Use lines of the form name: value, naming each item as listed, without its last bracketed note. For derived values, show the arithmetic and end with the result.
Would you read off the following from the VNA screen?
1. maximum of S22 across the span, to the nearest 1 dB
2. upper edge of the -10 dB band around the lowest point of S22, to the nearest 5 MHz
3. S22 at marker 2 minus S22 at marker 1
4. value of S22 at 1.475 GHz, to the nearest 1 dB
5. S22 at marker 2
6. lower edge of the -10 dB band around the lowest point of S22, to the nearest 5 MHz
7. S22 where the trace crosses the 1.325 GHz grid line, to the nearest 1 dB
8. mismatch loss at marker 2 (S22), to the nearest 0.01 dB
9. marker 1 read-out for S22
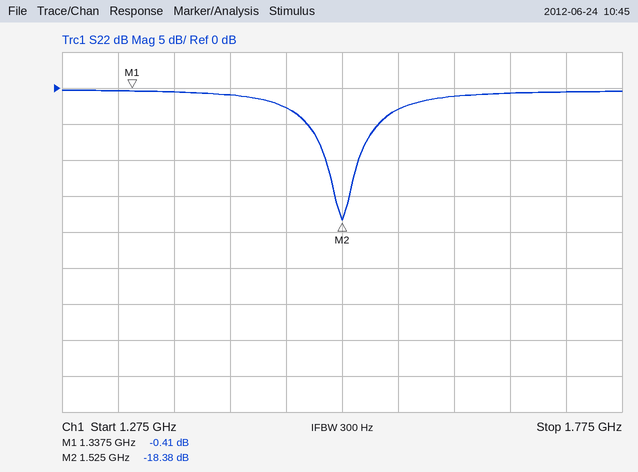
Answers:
maximum of S22 across the span, to the nearest 1 dB: 0 dB
upper edge of the -10 dB band around the lowest point of S22, to the nearest 5 MHz: 1.540 GHz
S22 at marker 2 minus S22 at marker 1: -18.38 − (-0.41) = -17.97 dB
value of S22 at 1.475 GHz, to the nearest 1 dB: -3 dB
S22 at marker 2: -18.38 dB
lower edge of the -10 dB band around the lowest point of S22, to the nearest 5 MHz: 1.510 GHz
S22 where the trace crosses the 1.325 GHz grid line, to the nearest 1 dB: 0 dB
mismatch loss at marker 2 (S22), to the nearest 0.01 dB: −10 log10(1 − 10^(-18.38/10)) ≈ 0.06 dB
marker 1 read-out for S22: -0.41 dB
